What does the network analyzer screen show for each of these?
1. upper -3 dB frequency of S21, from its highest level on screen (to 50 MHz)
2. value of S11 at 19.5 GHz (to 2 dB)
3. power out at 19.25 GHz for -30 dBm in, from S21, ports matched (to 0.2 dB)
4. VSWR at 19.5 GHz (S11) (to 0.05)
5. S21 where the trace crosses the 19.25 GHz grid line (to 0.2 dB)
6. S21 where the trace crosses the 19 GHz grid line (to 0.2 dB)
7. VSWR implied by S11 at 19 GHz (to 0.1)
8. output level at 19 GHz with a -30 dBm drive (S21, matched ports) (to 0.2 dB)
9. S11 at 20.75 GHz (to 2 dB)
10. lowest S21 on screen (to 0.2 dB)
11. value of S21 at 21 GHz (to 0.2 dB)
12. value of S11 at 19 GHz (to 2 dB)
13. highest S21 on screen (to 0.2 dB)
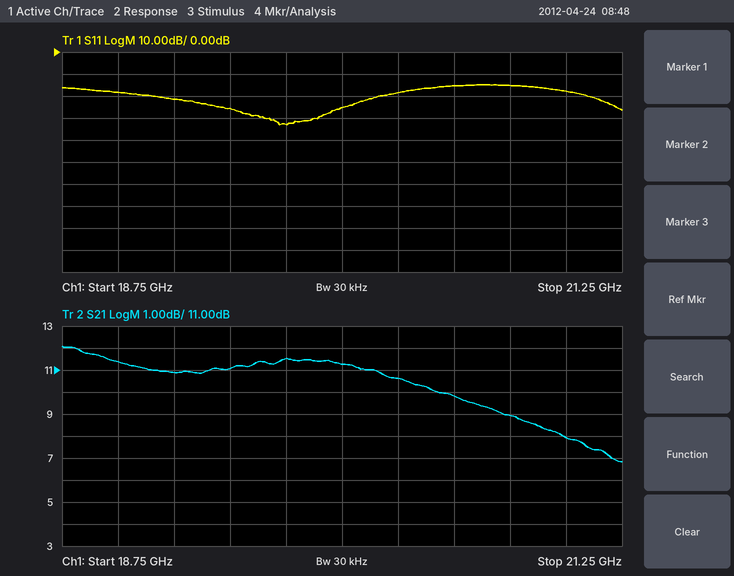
20.70 GHz
-26 dB
-19.2 dBm
1.10
10.8 dB
11.4 dB
1.3
-18.6 dBm
-16 dB
6.8 dB
8.0 dB
-18 dB
12.0 dB
